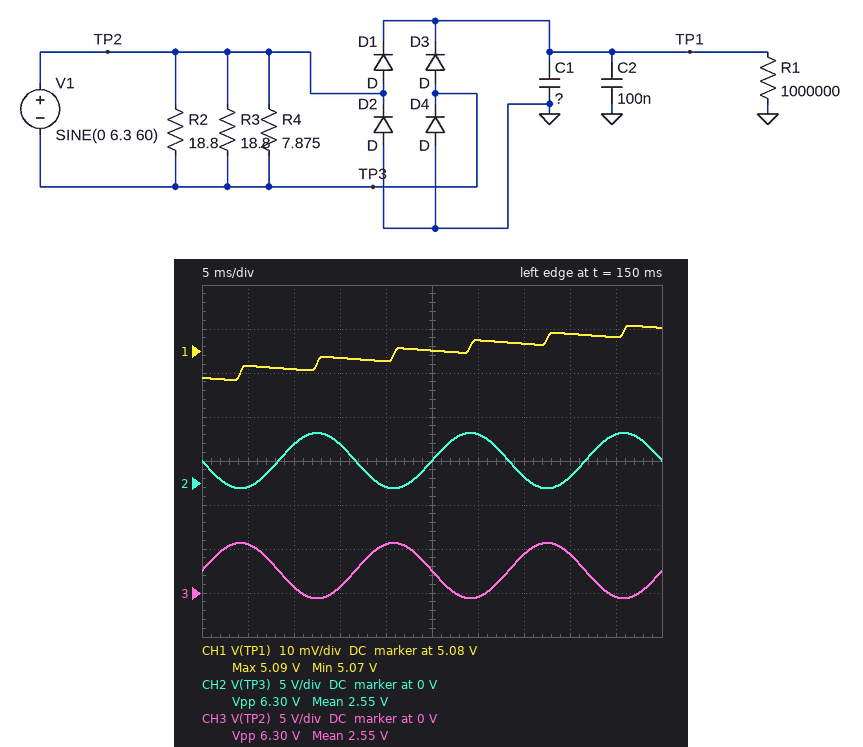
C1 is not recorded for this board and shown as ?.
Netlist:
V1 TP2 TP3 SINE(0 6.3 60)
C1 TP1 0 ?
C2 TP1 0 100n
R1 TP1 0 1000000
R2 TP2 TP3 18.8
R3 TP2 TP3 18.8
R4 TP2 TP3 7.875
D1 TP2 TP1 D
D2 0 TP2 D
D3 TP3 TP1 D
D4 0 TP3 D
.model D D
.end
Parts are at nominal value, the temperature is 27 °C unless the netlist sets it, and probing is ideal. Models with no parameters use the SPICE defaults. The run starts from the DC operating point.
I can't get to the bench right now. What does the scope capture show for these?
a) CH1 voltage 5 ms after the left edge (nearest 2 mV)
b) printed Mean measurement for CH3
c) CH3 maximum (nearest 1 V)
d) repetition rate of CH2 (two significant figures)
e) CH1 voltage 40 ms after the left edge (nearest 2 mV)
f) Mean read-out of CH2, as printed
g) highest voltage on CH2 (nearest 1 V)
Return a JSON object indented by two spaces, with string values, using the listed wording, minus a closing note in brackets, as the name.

{
  "CH1 voltage 5 ms after the left edge": "5.076 V",
  "printed Mean measurement for CH3": "2.55 V",
  "CH3 maximum": "6 V",
  "repetition rate of CH2": "60 Hz",
  "CH1 voltage 40 ms after the left edge": "5.084 V",
  "Mean read-out of CH2, as printed": "2.55 V",
  "highest voltage on CH2": "6 V"
}
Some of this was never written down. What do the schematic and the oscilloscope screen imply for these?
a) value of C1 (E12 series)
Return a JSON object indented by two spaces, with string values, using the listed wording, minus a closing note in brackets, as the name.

{
  "value of C1": "33 µF"
}
